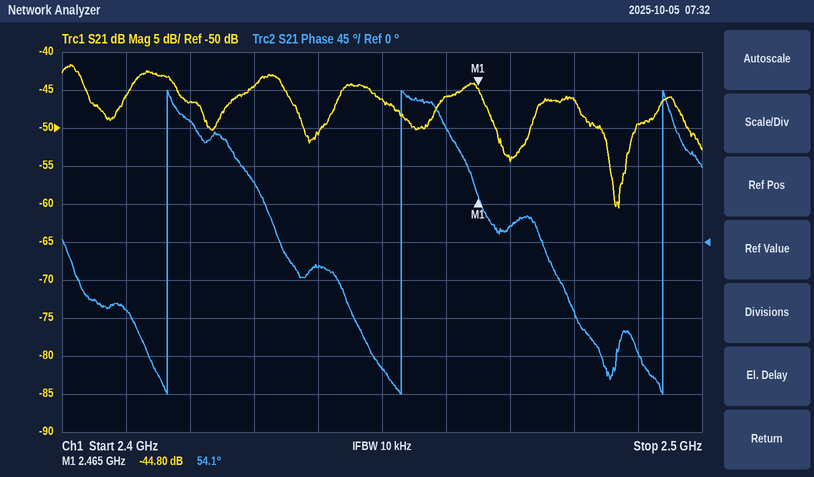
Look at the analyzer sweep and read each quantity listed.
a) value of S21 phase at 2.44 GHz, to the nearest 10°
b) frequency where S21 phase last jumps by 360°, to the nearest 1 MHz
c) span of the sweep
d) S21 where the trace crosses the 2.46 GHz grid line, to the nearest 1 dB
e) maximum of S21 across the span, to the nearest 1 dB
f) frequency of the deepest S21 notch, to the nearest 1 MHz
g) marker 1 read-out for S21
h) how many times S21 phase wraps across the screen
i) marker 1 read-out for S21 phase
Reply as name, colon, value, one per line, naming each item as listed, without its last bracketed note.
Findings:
value of S21 phase at 2.44 GHz, to the nearest 10°: -30°
frequency where S21 phase last jumps by 360°, to the nearest 1 MHz: 2.494 GHz
span of the sweep: 100 MHz
S21 where the trace crosses the 2.46 GHz grid line, to the nearest 1 dB: -46 dB
maximum of S21 across the span, to the nearest 1 dB: -42 dB
frequency of the deepest S21 notch, to the nearest 1 MHz: 2.487 GHz
marker 1 read-out for S21: -44.80 dB
how many times S21 phase wraps across the screen: 3
marker 1 read-out for S21 phase: 54.1°
